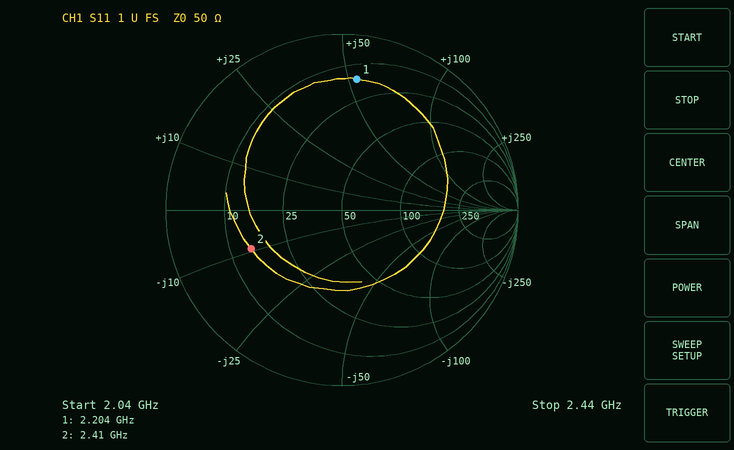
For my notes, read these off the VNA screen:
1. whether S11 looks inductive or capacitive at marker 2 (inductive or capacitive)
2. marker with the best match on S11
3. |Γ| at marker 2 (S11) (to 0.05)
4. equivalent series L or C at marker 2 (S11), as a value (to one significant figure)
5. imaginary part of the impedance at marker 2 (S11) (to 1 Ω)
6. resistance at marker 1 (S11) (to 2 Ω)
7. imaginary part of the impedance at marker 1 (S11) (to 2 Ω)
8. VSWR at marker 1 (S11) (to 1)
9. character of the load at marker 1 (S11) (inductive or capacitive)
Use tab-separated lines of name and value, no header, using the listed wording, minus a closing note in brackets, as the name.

whether S11 looks inductive or capacitive at marker 2	capacitive
marker with the best match on S11	marker 2
|Γ| at marker 2 (S11)	0.55
equivalent series L or C at marker 2 (S11), as a value	7 pF
imaginary part of the impedance at marker 2 (S11)	-9 Ω
resistance at marker 1 (S11)	16 Ω
imaginary part of the impedance at marker 1 (S11)	+54 Ω
VSWR at marker 1 (S11)	7
character of the load at marker 1 (S11)	inductive
